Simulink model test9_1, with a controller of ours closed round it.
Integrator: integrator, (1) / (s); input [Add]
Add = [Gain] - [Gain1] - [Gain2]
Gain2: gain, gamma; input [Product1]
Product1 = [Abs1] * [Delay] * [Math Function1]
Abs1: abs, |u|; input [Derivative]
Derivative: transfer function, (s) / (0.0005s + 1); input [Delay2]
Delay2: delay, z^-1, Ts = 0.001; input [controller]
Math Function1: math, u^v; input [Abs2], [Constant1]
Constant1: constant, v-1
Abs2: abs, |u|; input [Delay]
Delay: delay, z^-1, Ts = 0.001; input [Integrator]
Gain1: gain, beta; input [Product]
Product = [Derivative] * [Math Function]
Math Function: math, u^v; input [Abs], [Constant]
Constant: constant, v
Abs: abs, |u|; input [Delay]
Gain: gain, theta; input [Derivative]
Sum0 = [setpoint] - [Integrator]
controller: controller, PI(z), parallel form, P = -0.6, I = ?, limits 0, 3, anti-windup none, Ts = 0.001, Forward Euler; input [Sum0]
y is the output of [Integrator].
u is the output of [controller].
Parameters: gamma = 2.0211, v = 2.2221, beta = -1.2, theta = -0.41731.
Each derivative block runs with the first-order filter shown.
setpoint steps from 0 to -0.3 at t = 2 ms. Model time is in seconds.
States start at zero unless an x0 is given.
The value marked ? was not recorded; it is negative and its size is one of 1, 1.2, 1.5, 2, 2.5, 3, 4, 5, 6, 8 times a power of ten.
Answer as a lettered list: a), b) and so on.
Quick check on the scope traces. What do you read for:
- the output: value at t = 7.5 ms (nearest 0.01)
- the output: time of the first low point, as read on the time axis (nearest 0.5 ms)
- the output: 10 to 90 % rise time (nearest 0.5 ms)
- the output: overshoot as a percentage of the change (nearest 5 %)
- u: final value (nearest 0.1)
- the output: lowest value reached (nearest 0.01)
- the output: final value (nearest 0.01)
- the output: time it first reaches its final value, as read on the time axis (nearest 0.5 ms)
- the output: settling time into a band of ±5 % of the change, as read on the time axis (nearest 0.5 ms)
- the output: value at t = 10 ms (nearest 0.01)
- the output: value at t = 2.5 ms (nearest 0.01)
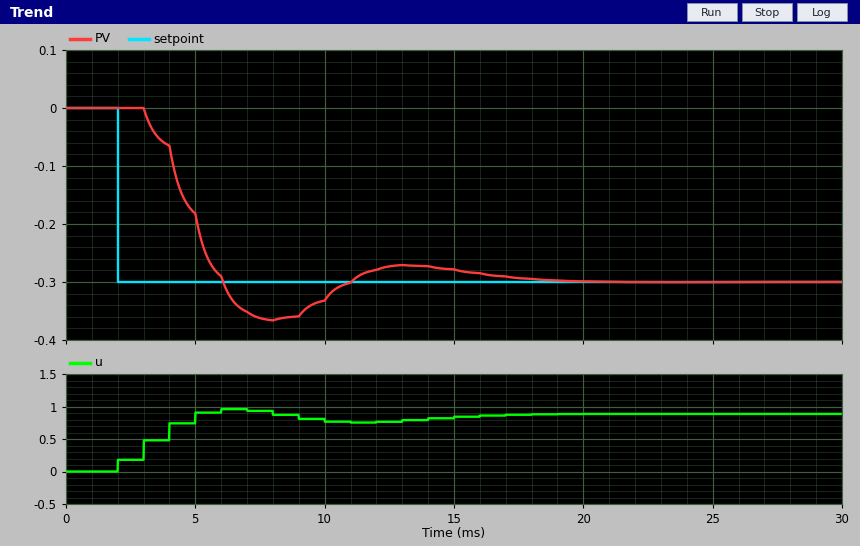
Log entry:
a) -0.36
b) 8.0 ms
c) 2.5 ms
d) 20 %
e) 0.9
f) -0.37
g) -0.30
h) 6.0 ms
i) 16.0 ms
j) -0.33
k) 0.00
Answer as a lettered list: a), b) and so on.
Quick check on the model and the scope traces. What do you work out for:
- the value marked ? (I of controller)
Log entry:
a) -1000
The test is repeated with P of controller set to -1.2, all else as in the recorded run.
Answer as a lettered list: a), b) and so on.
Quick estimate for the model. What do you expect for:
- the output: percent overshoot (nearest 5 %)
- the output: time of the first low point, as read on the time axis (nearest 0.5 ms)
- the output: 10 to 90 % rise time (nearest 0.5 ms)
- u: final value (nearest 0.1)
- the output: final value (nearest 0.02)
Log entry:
a) 10 %
b) 7.0 ms
c) 2.0 ms
d) 0.8
e) -0.30
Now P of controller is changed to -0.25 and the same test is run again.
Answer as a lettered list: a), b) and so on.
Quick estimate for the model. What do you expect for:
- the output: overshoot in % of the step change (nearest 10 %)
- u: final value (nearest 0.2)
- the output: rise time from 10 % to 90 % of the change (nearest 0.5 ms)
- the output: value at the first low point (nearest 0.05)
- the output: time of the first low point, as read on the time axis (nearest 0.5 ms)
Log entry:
a) 30 %
b) 1.0
c) 2.0 ms
d) -0.40
e) 9.0 ms
